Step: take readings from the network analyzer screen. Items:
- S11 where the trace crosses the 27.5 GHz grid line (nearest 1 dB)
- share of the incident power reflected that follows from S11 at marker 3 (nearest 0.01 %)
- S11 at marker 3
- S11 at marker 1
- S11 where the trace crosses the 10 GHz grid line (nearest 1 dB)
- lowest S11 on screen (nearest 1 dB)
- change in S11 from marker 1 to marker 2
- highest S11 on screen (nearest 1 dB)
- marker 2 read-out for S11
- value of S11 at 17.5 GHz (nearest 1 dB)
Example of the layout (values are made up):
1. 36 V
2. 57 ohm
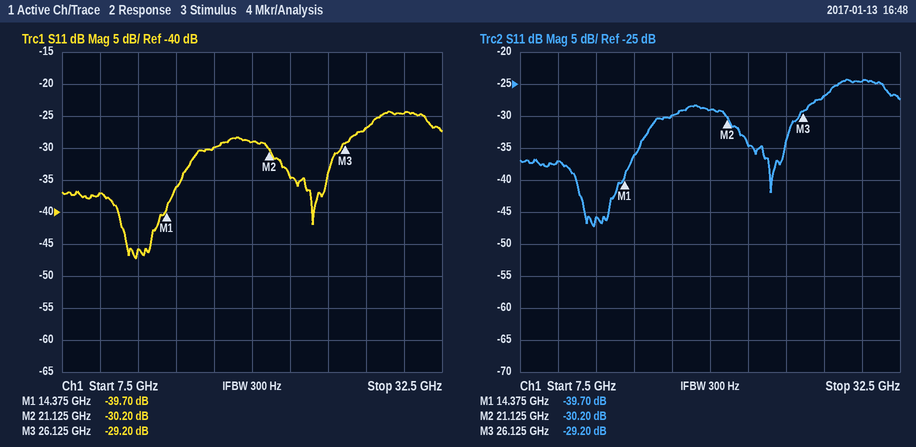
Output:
1. -27 dB
2. 0.12 %
3. -29.20 dB
4. -39.70 dB
5. -37 dB
6. -47 dB
7. 9.50 dB
8. -24 dB
9. -30.20 dB
10. -30 dB
